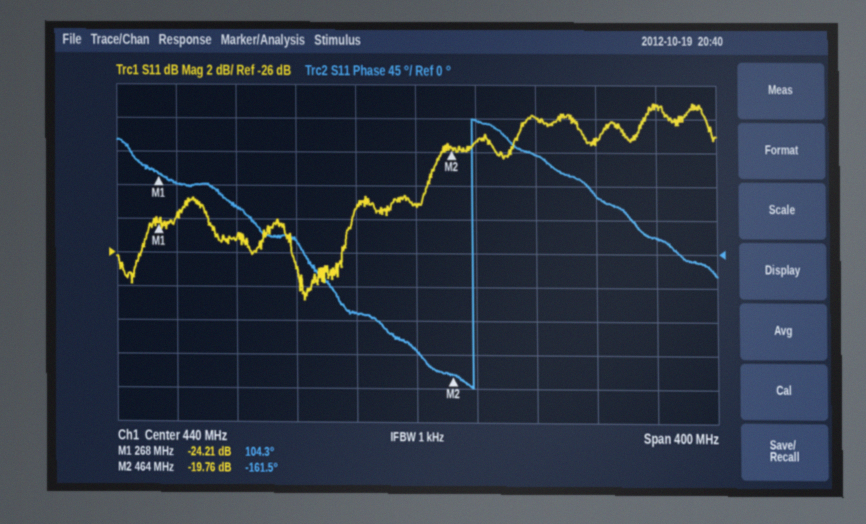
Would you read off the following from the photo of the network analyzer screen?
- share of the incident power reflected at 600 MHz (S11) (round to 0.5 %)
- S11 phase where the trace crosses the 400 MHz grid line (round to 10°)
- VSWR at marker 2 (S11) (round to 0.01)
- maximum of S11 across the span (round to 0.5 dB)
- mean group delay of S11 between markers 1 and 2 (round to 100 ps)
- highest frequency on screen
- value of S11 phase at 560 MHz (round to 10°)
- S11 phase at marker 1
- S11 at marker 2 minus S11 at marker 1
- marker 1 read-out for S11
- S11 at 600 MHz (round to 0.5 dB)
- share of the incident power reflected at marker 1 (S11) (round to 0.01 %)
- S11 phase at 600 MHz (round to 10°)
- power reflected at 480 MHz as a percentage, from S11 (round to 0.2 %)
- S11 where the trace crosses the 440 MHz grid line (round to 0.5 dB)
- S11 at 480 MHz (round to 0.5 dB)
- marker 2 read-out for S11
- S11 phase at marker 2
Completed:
2.0 %
-80°
1.23
-17.0 dB
3.8 ns
640 MHz
80°
104.3°
4.45 dB
-24.21 dB
-17.0 dB
0.38 %
20°
1.2 %
-23.0 dB
-19.5 dB
-19.76 dB
-161.5°
